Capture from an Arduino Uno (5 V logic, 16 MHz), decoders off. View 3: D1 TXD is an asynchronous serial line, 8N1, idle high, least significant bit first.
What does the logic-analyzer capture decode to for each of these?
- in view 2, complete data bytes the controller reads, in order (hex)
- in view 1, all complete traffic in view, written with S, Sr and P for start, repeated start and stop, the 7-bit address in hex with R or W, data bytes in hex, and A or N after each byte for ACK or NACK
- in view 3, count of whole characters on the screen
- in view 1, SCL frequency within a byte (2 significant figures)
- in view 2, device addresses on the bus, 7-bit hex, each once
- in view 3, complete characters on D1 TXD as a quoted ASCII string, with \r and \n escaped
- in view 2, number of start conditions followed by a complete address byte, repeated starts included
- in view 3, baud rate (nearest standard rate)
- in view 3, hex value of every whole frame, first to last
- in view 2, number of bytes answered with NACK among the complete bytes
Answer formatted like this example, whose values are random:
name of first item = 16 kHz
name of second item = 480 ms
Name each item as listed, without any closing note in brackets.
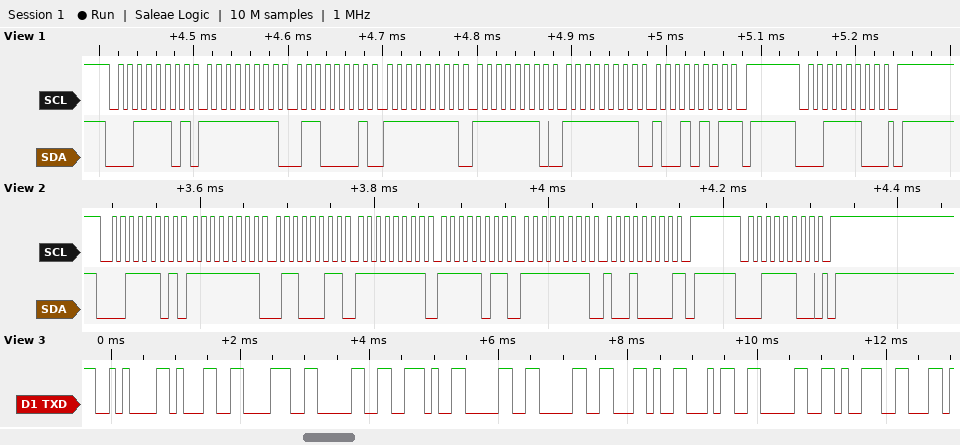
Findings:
in view 2, complete data bytes the controller reads, in order = FF 63 FF FB FF 90
in view 1, all complete traffic in view, written with S, Sr and P for start, repeated start and stop, the 7-bit address in hex with R or W, data bytes in hex, and A or N after each byte for ACK or NACK = S 1ER A FF A 61 A FF A FE A FF A 95 N P S 1EW A P
in view 3, count of whole characters on the screen = 11
in view 1, SCL frequency within a byte = 100 kHz
in view 2, device addresses on the bus, 7-bit hex, each once = 0x1E
in view 3, complete characters on D1 TXD as a quoted ASCII string, with \r and \n escaped = "\n180.00,409"
in view 2, number of start conditions followed by a complete address byte, repeated starts included = 2
in view 3, baud rate = 9600 baud
in view 3, hex value of every whole frame, first to last = 0A 31 38 30 2E 30 30 2C 34 30 39
in view 2, number of bytes answered with NACK among the complete bytes = 1
